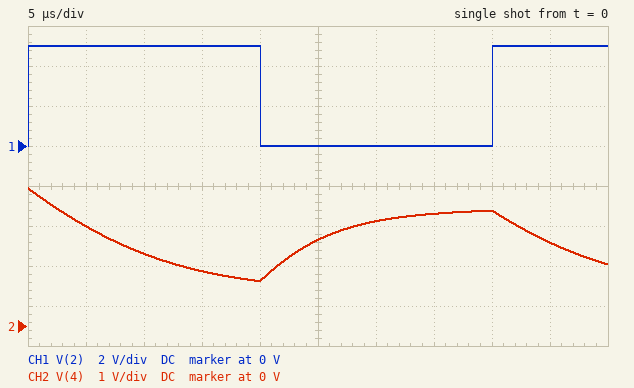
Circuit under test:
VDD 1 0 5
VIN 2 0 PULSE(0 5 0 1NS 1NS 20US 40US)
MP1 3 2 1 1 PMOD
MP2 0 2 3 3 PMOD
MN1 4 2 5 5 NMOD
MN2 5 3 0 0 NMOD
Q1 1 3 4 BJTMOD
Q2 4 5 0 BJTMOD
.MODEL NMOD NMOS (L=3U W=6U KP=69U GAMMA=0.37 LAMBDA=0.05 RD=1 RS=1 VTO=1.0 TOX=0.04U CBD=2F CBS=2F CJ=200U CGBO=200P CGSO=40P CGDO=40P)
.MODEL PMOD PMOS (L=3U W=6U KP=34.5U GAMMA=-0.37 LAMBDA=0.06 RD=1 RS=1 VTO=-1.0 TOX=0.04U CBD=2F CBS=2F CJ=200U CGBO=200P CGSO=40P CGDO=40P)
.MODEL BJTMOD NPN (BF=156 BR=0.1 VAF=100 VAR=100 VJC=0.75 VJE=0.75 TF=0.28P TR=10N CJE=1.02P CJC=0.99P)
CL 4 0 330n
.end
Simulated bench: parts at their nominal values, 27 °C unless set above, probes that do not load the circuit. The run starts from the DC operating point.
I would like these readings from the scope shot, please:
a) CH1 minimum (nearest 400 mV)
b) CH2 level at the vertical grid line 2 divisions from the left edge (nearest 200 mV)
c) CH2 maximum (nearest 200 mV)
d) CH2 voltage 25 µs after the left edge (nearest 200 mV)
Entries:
0 V
1.8 V
3.4 V
2.2 V
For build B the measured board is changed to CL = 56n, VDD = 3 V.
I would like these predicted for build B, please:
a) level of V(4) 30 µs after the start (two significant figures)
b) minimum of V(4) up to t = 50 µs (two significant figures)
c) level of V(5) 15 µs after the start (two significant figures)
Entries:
1.6 V
740 mV
730 mV
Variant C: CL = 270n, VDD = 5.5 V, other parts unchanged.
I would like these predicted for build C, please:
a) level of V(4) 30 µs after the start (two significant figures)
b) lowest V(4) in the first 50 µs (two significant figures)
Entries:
3.1 V
1.0 V
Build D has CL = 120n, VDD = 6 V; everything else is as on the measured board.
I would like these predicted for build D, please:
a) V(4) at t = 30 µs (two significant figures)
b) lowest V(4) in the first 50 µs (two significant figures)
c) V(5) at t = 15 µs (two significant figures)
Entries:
3.6 V
800 mV
790 mV
